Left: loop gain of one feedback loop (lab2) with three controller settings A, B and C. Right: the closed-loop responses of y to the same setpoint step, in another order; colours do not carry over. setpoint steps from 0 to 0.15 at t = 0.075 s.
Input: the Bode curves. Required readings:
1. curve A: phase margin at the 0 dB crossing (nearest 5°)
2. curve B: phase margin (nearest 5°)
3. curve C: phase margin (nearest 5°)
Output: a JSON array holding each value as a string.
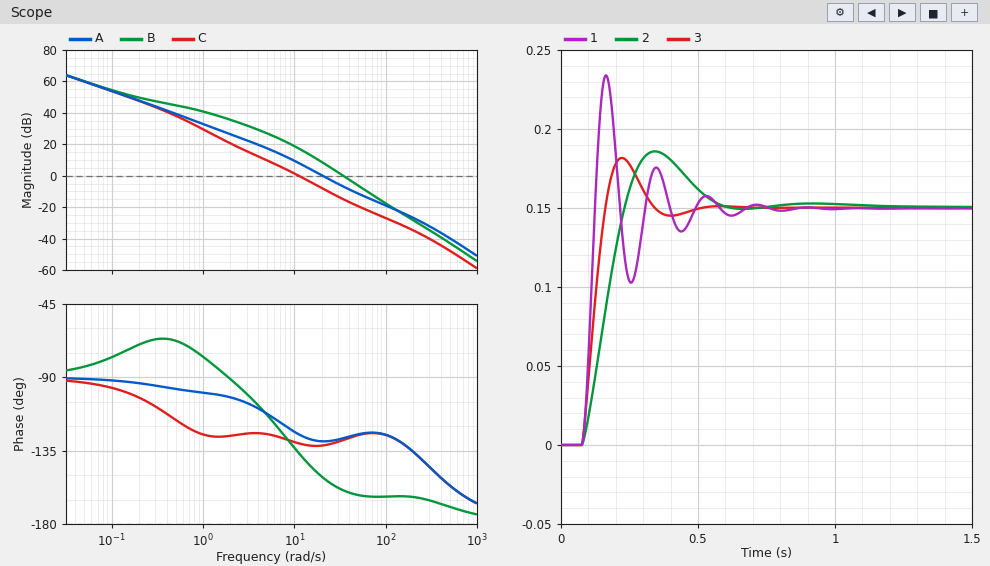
["50°", "20°", "50°"]
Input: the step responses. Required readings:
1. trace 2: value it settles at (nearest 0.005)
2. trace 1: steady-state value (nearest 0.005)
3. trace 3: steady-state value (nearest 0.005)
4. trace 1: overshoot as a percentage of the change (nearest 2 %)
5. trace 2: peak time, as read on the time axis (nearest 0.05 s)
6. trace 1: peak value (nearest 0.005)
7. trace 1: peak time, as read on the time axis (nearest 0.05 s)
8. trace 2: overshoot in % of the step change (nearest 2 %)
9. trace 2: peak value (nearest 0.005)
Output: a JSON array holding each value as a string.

["0.150", "0.150", "0.150", "56 %", "0.35 s", "0.235", "0.15 s", "24 %", "0.185"]
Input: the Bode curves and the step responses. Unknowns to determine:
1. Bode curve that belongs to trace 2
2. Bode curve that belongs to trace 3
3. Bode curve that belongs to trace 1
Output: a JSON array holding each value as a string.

["C", "A", "B"]
